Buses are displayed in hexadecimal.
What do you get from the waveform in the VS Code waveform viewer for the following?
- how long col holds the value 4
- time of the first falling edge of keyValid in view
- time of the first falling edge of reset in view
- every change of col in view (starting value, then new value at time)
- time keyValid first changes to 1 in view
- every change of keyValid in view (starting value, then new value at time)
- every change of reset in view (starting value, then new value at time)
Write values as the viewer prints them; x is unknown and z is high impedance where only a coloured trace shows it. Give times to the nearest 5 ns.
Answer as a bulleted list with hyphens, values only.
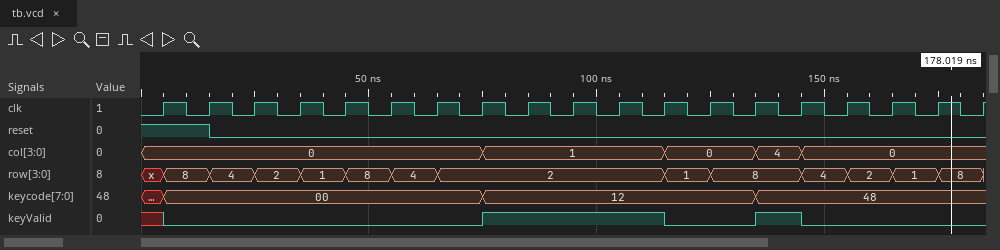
- 10 ns
- 115 ns
- 15 ns
- 0, 1 at 75 ns, 0 at 115 ns, 4 at 135 ns, 0 at 145 ns
- 75 ns
- x, 0 at 5 ns, 1 at 75 ns, 0 at 115 ns, 1 at 135 ns, 0 at 145 ns
- 1, 0 at 15 ns
